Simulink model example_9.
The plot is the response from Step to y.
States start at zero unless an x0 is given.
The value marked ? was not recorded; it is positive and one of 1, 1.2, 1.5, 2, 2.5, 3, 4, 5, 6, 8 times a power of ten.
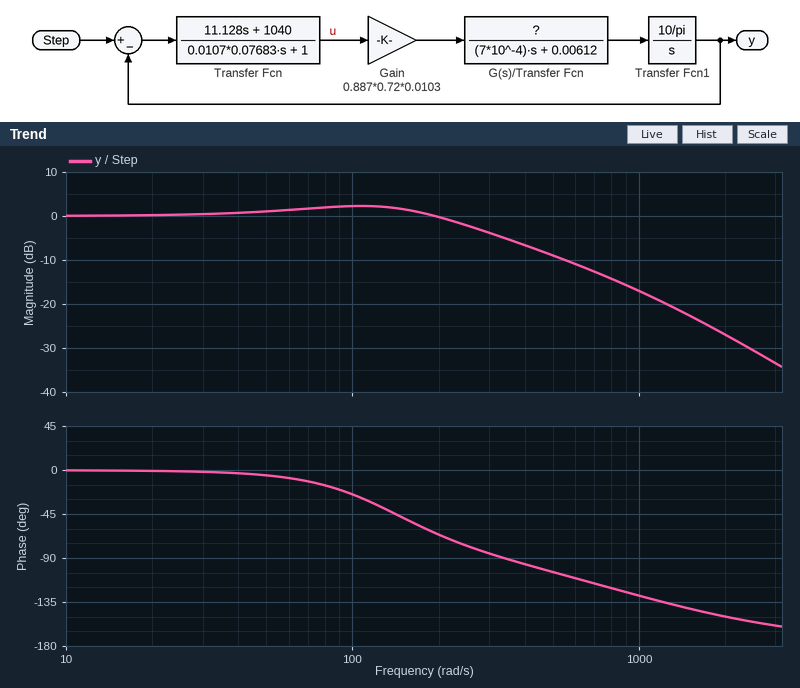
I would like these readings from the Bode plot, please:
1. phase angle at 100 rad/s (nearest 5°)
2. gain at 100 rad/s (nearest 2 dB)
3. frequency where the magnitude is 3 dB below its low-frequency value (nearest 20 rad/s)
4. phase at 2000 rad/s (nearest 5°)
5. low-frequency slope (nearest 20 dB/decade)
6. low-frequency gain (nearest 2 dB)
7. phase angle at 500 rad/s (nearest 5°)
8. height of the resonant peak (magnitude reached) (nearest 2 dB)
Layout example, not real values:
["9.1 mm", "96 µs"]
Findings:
["-25°", "2 dB", "280 rad/s", "-150°", "0 dB/decade", "0 dB", "-105°", "2 dB"]
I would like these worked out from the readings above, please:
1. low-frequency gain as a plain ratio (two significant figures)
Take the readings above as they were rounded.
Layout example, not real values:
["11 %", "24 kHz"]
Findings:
["1.0"]
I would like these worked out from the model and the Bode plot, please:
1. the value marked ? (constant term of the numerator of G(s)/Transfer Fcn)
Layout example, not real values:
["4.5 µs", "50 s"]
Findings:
["0.5"]
